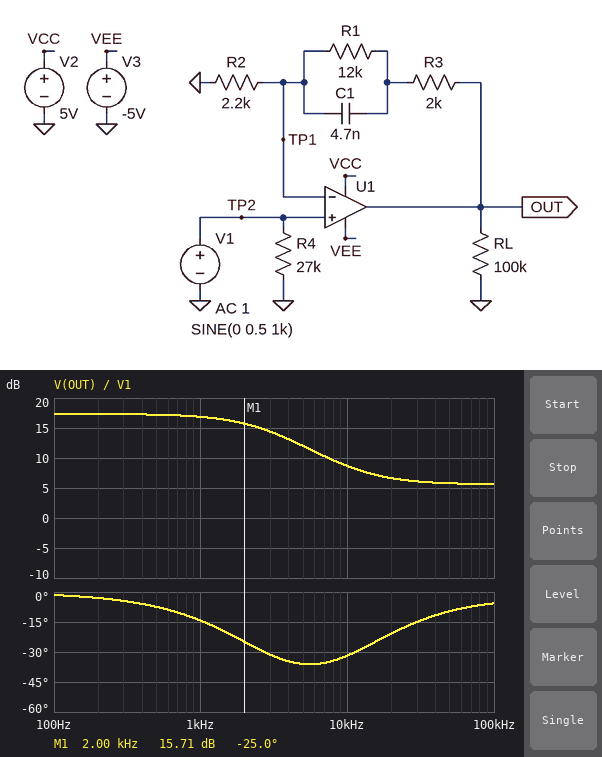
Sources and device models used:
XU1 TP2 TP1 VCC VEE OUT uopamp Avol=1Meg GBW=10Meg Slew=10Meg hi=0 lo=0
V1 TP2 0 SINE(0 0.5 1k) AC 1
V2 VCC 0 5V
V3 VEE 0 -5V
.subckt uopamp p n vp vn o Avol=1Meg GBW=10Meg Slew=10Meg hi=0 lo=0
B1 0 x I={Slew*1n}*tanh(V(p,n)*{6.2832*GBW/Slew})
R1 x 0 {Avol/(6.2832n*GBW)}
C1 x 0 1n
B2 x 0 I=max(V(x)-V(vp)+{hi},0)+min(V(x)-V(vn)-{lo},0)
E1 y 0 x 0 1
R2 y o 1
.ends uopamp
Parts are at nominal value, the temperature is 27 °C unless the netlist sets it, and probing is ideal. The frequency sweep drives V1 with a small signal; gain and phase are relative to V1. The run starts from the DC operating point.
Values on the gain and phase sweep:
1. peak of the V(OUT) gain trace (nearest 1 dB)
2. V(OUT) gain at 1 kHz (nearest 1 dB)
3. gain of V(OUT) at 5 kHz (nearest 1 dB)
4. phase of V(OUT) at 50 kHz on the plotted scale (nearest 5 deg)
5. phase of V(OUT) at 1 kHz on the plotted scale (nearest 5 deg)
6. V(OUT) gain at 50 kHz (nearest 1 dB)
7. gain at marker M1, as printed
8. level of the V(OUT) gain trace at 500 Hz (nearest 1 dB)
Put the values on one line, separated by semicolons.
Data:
17 dB; 17 dB; 12 dB; -10 deg; -15 deg; 6 dB; 15.71 dB; 17 dB
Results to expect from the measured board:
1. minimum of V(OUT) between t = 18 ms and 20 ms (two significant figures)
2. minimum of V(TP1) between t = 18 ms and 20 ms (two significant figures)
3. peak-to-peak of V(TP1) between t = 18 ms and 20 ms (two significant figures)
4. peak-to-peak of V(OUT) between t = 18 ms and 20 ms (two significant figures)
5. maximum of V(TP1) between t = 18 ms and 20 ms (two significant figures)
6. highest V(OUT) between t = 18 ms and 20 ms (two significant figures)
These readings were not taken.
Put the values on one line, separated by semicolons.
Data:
-3.5 V; -500 mV; 1.0 V; 7.0 V; 500 mV; 3.5 V
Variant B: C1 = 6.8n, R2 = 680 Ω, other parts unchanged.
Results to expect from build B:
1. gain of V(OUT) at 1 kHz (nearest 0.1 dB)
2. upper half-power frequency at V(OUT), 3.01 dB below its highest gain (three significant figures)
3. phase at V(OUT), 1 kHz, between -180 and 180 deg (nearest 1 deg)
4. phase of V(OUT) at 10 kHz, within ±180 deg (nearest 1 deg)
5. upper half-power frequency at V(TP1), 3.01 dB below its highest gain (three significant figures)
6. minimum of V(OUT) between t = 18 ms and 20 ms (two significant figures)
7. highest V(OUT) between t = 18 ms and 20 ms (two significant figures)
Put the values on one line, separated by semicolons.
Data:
25.7 dB; 2.01 kHz; -22 deg; -36 deg; 2.53 MHz; -5.0 V; 5.0 V
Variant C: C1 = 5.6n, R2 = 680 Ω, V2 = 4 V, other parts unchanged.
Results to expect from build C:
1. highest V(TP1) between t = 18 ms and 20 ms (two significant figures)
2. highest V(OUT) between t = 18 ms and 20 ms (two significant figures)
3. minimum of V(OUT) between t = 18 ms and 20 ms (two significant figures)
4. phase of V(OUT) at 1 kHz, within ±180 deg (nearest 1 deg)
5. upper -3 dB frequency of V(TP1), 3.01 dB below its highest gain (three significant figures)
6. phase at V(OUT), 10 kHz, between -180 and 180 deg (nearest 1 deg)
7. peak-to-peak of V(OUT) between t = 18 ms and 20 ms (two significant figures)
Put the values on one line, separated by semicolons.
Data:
330 mV; 4.0 V; -5.0 V; -19 deg; 2.53 MHz; -39 deg; 9.0 V
